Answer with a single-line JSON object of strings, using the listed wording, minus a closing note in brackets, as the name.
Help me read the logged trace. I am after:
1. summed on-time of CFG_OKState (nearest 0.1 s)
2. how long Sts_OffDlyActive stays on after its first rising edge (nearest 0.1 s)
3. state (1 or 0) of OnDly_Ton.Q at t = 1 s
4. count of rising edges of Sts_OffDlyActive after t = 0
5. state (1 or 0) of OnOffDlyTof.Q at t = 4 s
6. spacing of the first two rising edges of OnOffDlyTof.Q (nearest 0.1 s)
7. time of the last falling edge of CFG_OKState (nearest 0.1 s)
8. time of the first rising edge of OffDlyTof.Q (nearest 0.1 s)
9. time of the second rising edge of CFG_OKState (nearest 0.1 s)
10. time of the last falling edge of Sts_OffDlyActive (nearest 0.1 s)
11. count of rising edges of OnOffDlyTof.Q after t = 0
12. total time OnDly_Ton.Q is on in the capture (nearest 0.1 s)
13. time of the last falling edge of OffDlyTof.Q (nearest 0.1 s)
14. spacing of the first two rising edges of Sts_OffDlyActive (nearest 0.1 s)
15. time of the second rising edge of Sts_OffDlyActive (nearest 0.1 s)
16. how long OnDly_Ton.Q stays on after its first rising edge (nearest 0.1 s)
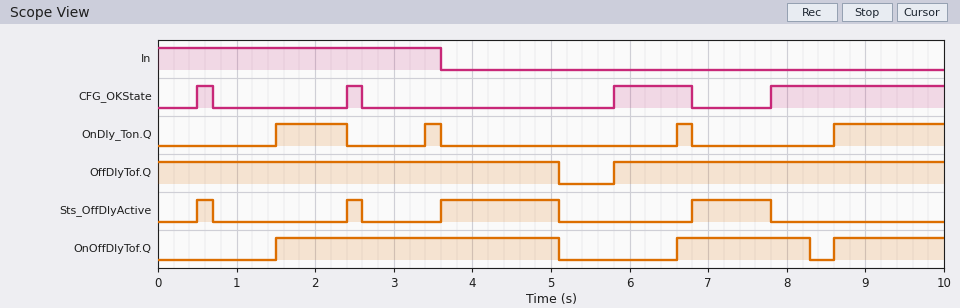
{"summed on-time of CFG_OKState": "3.6 s", "how long Sts_OffDlyActive stays on after its first rising edge": "0.2 s", "state (1 or 0) of OnDly_Ton.Q at t = 1 s": "0", "count of rising edges of Sts_OffDlyActive after t = 0": "4", "state (1 or 0) of OnOffDlyTof.Q at t = 4 s": "1", "spacing of the first two rising edges of OnOffDlyTof.Q": "5.1 s", "time of the last falling edge of CFG_OKState": "6.8 s", "time of the first rising edge of OffDlyTof.Q": "5.8 s", "time of the second rising edge of CFG_OKState": "2.4 s", "time of the last falling edge of Sts_OffDlyActive": "7.8 s", "count of rising edges of OnOffDlyTof.Q after t = 0": "3", "total time OnDly_Ton.Q is on in the capture": "2.7 s", "time of the last falling edge of OffDlyTof.Q": "5.1 s", "spacing of the first two rising edges of Sts_OffDlyActive": "1.9 s", "time of the second rising edge of Sts_OffDlyActive": "2.4 s", "how long OnDly_Ton.Q stays on after its first rising edge": "0.9 s"}
